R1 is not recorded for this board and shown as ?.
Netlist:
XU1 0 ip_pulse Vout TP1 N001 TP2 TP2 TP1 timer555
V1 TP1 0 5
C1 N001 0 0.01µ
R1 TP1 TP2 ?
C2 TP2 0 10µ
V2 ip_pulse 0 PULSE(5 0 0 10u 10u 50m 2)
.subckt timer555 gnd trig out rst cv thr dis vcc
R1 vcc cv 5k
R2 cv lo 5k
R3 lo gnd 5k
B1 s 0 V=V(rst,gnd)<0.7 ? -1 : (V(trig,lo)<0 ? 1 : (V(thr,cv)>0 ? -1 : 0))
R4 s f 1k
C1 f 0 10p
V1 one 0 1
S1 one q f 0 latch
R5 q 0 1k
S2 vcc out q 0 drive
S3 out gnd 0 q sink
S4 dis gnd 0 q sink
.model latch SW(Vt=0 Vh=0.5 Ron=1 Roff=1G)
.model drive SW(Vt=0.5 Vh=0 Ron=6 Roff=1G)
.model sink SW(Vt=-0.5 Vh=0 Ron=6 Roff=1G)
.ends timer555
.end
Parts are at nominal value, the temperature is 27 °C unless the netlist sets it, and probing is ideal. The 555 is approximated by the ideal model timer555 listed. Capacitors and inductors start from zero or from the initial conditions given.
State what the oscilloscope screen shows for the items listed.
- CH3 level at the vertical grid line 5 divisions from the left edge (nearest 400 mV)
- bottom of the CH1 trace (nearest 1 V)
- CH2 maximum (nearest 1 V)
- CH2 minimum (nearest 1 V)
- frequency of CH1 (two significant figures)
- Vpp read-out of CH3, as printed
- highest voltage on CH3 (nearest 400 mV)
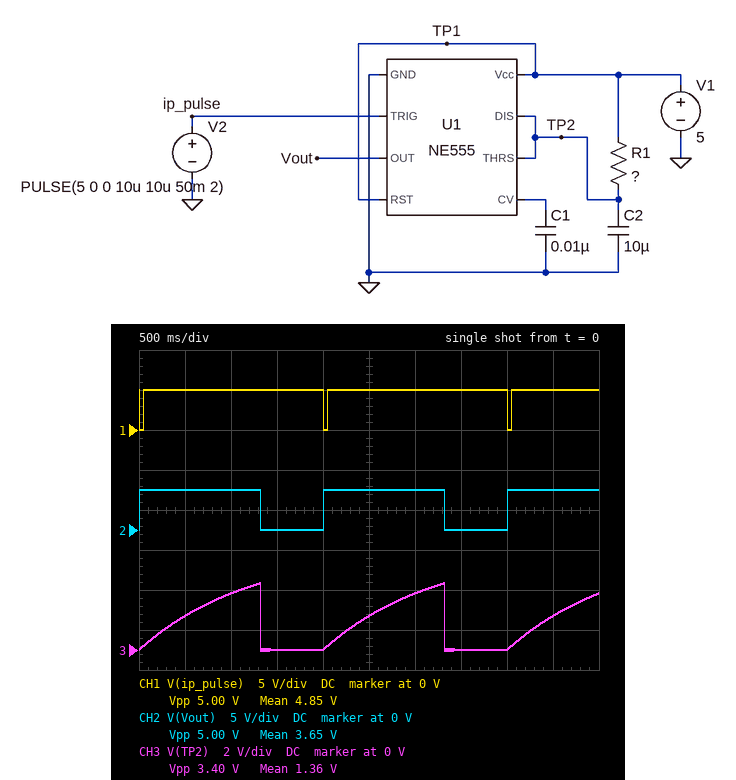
1.6 V
0 V
5 V
0 V
500 mHz
3.40 V
3.2 V
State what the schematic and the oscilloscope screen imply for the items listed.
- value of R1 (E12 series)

120 kΩ
